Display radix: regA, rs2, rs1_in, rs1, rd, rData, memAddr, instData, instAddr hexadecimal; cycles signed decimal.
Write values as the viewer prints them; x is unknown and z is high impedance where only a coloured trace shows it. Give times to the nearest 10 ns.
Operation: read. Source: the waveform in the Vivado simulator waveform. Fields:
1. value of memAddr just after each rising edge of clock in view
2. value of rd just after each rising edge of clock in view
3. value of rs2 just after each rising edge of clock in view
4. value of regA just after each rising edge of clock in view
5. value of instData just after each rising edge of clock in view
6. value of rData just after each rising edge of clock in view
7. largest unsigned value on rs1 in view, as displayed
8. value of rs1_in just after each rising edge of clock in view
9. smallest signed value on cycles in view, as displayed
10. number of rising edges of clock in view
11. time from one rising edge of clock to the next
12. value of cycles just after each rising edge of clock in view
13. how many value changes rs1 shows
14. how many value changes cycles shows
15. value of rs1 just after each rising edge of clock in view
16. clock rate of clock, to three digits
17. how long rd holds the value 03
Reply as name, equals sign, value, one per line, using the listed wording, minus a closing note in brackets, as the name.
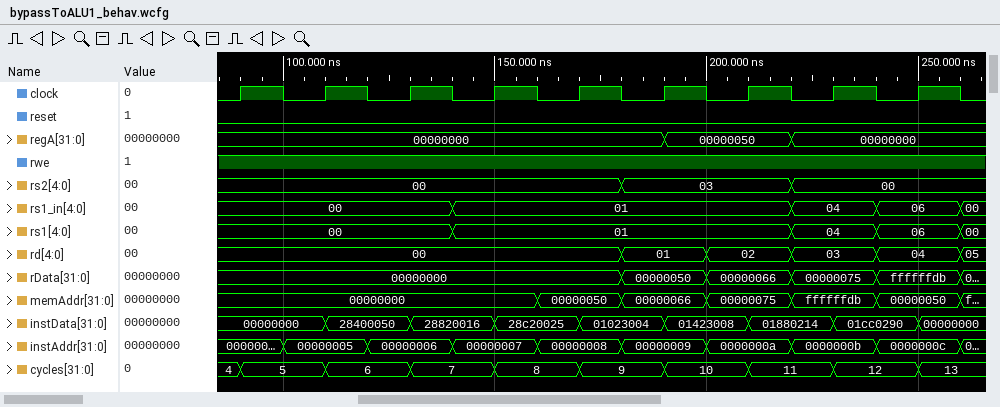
value of memAddr just after each rising edge of clock in view = 00000000, 00000000, 00000000, 00000000, 00000050, 00000066, 00000075, ffffffdb, 00000050
value of rd just after each rising edge of clock in view = 00, 00, 00, 00, 00, 01, 02, 03, 04
value of rs2 just after each rising edge of clock in view = 00, 00, 00, 00, 00, 03, 03, 00, 00
value of regA just after each rising edge of clock in view = 00000000, 00000000, 00000000, 00000000, 00000000, 00000050, 00000050, 00000000, 00000000
value of instData just after each rising edge of clock in view = 00000000, 28400050, 28820016, 28c20025, 01023004, 01423008, 01880214, 01cc0290, 00000000
value of rData just after each rising edge of clock in view = 00000000, 00000000, 00000000, 00000000, 00000000, 00000050, 00000066, 00000075, ffffffdb
largest unsigned value on rs1 in view, as displayed = 06
value of rs1_in just after each rising edge of clock in view = 00, 00, 00, 01, 01, 01, 01, 04, 06
smallest signed value on cycles in view, as displayed = 4
number of rising edges of clock in view = 9
time from one rising edge of clock to the next = 20 ns
value of cycles just after each rising edge of clock in view = 5, 6, 7, 8, 9, 10, 11, 12, 13
how many value changes rs1 shows = 4
how many value changes cycles shows = 9
value of rs1 just after each rising edge of clock in view = 00, 00, 00, 01, 01, 01, 01, 04, 06
clock rate of clock, to three digits = 50.0 MHz
how long rd holds the value 03 = 20 ns
